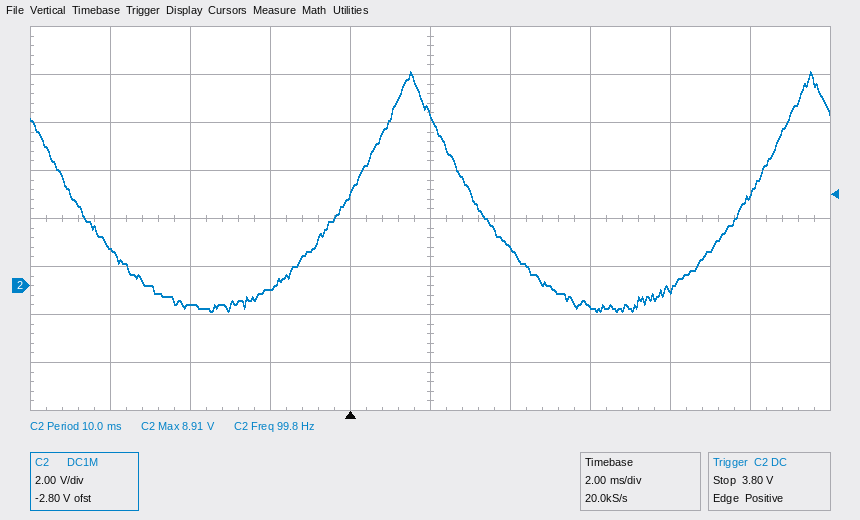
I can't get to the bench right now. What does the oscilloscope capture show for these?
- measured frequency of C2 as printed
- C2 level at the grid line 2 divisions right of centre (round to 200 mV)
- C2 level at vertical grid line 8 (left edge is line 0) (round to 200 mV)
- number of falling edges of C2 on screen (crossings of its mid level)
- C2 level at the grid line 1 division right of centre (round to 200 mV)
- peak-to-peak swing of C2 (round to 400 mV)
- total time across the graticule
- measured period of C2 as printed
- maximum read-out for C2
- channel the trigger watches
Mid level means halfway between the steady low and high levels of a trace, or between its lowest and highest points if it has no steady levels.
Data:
99.8 Hz
-800 mV
-200 mV
2
1.6 V
10.0 V
20 ms
10.0 ms
8.91 V
C2
